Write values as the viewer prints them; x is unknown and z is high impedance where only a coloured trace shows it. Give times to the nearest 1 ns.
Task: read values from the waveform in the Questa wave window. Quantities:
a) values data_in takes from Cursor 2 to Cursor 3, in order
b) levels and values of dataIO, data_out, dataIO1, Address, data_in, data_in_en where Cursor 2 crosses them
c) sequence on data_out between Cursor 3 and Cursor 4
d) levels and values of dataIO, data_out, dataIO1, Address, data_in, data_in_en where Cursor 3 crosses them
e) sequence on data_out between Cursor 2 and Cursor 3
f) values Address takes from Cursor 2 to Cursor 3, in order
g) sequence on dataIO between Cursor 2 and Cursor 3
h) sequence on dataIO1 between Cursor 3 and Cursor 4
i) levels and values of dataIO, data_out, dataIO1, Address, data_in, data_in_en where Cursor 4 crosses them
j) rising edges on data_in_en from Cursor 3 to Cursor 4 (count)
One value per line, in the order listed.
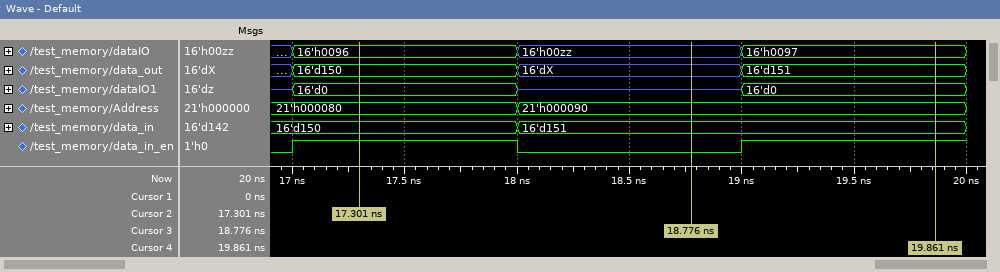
16'd150, 16'd151
dataIO=16'h0096, data_out=16'd150, dataIO1=16'd0, Address=21'h000080, data_in=16'd150, data_in_en=1
16'dX, 16'd151
dataIO=16'h00zz, data_out=16'dX, dataIO1=z, Address=21'h000090, data_in=16'd151, data_in_en=0
16'd150, 16'dX
21'h000080, 21'h000090
16'h0096, 16'h00zz
z, 16'd0
dataIO=16'h0097, data_out=16'd151, dataIO1=16'd0, Address=21'h000090, data_in=16'd151, data_in_en=1
1
